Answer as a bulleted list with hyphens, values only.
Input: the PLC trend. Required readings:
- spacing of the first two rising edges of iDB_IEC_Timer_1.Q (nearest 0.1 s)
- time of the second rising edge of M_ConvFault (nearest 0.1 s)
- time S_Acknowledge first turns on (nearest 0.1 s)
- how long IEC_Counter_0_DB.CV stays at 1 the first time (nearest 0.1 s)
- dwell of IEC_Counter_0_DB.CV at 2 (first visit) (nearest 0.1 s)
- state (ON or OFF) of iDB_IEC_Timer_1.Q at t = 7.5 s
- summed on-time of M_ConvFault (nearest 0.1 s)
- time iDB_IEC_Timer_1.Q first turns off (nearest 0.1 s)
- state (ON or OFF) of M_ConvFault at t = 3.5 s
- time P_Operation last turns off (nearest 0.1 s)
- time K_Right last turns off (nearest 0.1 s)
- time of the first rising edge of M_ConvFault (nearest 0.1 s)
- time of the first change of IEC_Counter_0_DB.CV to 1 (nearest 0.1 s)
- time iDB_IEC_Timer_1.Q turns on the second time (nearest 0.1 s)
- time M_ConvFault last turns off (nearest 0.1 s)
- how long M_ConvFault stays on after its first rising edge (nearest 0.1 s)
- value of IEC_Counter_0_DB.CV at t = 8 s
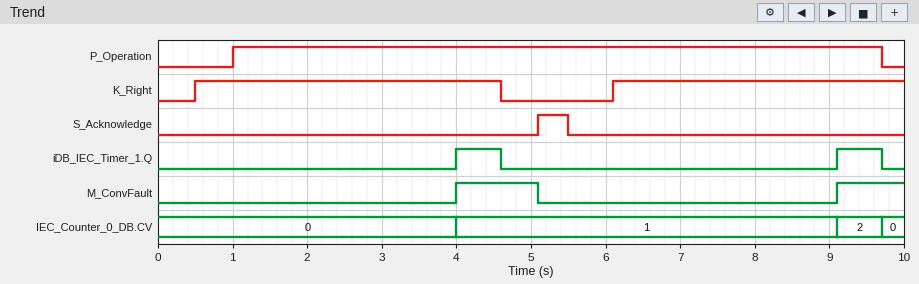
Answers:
- 5.1 s
- 9.1 s
- 5.1 s
- 5.1 s
- 0.6 s
- OFF
- 2.0 s
- 4.6 s
- OFF
- 9.7 s
- 4.6 s
- 4.0 s
- 4.0 s
- 9.1 s
- 5.1 s
- 1.1 s
- 1
